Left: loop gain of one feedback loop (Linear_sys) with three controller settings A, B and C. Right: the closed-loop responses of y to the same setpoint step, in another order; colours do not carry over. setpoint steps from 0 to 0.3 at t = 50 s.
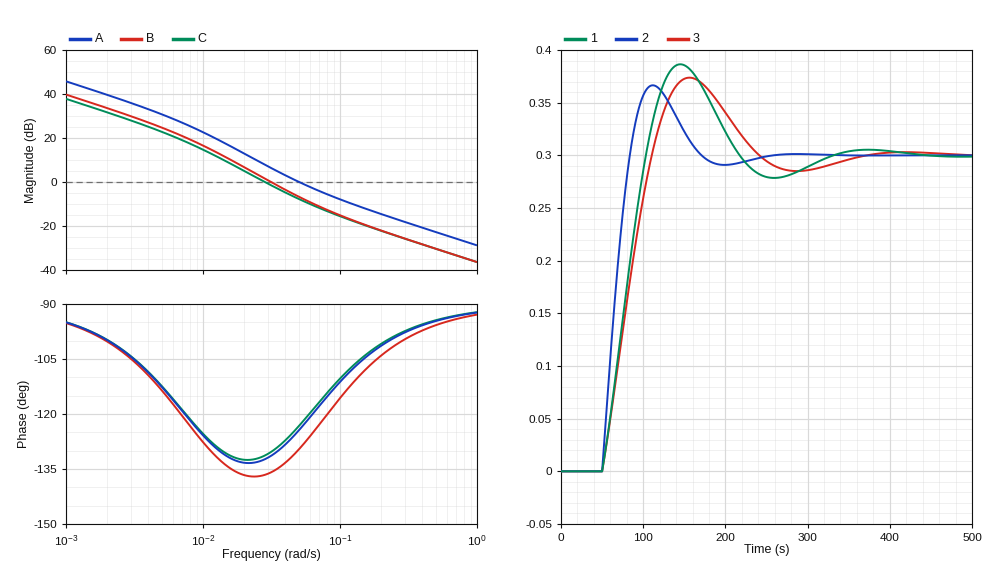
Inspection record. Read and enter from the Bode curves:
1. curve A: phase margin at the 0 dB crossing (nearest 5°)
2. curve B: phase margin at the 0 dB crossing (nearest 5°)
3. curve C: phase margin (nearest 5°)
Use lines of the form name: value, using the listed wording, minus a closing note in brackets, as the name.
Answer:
curve A: phase margin at the 0 dB crossing: 55°
curve B: phase margin at the 0 dB crossing: 45°
curve C: phase margin: 50°
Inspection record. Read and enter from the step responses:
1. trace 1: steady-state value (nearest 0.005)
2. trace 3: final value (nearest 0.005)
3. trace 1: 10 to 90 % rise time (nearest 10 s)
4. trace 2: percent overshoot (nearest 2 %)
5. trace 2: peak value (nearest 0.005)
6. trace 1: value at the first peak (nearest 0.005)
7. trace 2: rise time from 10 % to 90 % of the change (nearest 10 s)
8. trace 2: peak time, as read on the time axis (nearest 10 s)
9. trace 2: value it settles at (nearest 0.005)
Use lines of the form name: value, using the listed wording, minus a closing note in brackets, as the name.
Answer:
trace 1: steady-state value: 0.300
trace 3: final value: 0.300
trace 1: 10 to 90 % rise time: 40 s
trace 2: percent overshoot: 22 %
trace 2: peak value: 0.365
trace 1: value at the first peak: 0.385
trace 2: rise time from 10 % to 90 % of the change: 30 s
trace 2: peak time, as read on the time axis: 110 s
trace 2: value it settles at: 0.300
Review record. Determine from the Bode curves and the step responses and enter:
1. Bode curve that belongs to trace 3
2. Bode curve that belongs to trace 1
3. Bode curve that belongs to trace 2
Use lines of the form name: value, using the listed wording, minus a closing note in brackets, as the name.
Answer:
Bode curve that belongs to trace 3: C
Bode curve that belongs to trace 1: B
Bode curve that belongs to trace 2: A
